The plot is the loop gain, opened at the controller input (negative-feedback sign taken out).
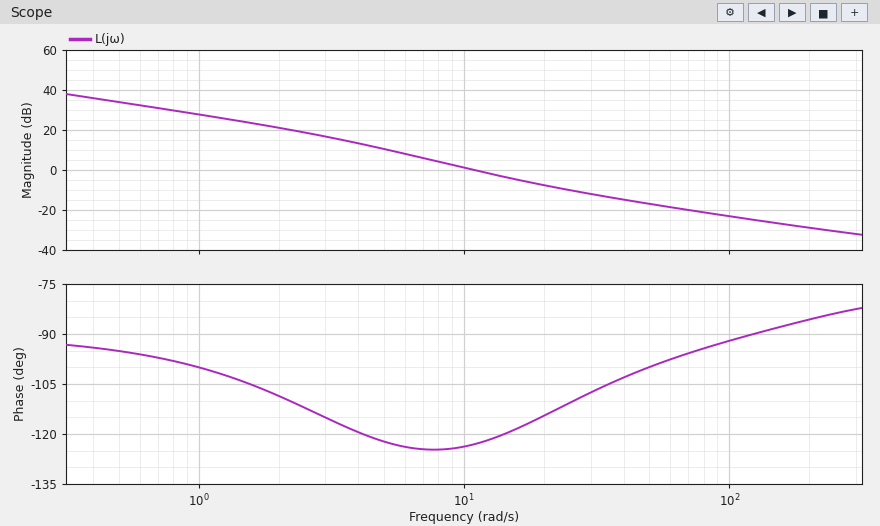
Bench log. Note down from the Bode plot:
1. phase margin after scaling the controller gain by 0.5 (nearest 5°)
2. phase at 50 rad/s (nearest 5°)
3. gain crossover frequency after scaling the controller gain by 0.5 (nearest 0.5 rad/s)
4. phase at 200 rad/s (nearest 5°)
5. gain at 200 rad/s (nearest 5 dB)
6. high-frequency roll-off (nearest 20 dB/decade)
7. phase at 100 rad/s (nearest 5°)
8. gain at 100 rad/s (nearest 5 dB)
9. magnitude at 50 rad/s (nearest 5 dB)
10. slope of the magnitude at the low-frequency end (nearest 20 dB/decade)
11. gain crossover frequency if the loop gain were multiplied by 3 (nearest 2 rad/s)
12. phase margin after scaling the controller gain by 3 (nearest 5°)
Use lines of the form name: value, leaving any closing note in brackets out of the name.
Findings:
phase margin after scaling the controller gain by 0.5: 55°
phase at 50 rad/s: -100°
gain crossover frequency after scaling the controller gain by 0.5: 7.0 rad/s
phase at 200 rad/s: -85°
gain at 200 rad/s: -30 dB
high-frequency roll-off: -20 dB/decade
phase at 100 rad/s: -90°
gain at 100 rad/s: -25 dB
magnitude at 50 rad/s: -15 dB
slope of the magnitude at the low-frequency end: -20 dB/decade
gain crossover frequency if the loop gain were multiplied by 3: 24 rad/s
phase margin after scaling the controller gain by 3: 70°
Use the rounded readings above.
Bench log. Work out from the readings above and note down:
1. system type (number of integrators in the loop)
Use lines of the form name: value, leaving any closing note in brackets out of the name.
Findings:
system type: 1
